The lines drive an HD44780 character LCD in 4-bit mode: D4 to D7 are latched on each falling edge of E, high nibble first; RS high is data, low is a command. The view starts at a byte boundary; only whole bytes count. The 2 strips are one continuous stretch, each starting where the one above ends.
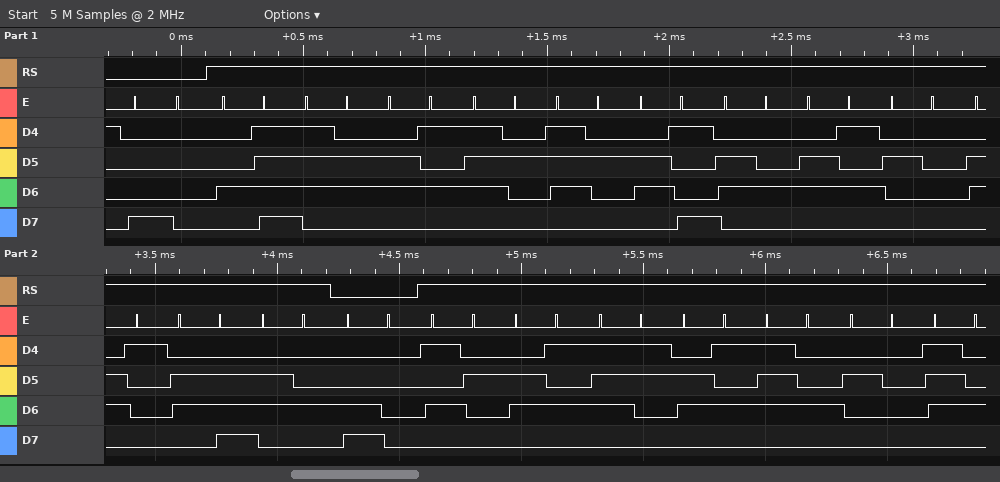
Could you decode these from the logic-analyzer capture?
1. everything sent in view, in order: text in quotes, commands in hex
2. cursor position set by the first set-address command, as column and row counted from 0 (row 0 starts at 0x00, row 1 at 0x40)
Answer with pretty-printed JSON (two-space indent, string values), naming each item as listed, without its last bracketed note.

{
  "everything sent in view, in order: text in quotes, commands in hex": "0x80 \"Override and\" 0xC0 \"Reset t\"",
  "cursor position set by the first set-address command, as column and row counted from 0": "column 0, row 0"
}
